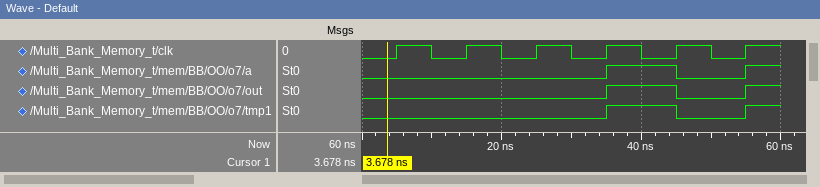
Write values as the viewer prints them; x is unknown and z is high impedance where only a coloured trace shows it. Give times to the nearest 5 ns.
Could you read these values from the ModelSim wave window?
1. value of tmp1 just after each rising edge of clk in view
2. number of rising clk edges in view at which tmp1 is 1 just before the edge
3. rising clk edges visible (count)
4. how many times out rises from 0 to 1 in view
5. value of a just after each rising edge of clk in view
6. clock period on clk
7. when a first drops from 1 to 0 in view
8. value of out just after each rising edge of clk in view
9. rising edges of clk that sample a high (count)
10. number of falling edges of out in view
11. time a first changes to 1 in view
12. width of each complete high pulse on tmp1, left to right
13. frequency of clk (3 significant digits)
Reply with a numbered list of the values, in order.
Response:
1. 0 0 0 1 0 1
2. 1
3. 6
4. 2
5. 0 0 0 1 0 1
6. 10 ns
7. 45 ns
8. 0 0 0 1 0 1
9. 1
10. 1
11. 35 ns
12. 10 ns
13. 100 MHz
